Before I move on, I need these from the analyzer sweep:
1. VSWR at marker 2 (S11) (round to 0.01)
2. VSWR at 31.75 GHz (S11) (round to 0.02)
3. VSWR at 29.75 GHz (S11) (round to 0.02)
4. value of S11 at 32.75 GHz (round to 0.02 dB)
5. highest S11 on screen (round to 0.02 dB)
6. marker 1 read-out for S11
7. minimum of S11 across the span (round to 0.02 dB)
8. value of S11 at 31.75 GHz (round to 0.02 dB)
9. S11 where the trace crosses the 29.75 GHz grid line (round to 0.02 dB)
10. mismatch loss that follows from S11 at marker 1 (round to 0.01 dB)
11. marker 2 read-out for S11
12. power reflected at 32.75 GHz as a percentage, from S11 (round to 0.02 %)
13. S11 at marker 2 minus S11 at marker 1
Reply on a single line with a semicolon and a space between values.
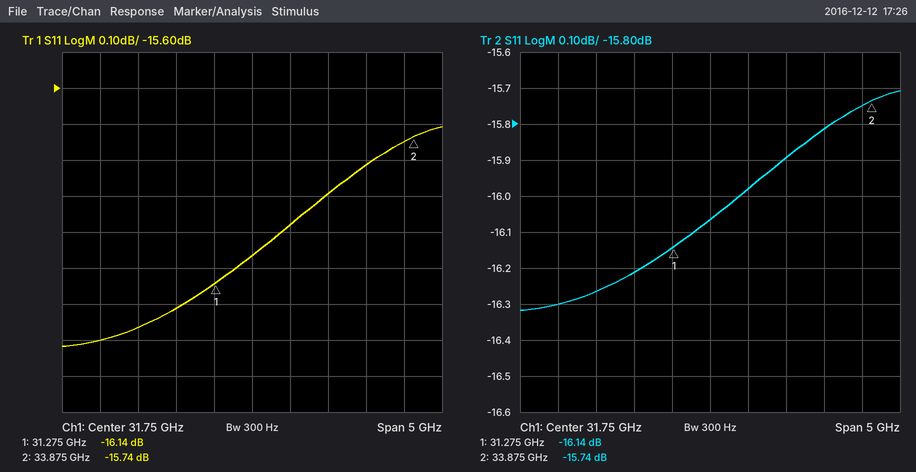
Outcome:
1.39; 1.38; 1.36; -15.90 dB; -15.70 dB; -16.14 dB; -16.32 dB; -16.06 dB; -16.30 dB; 0.11 dB; -15.74 dB; 2.58 %; 0.40 dB
